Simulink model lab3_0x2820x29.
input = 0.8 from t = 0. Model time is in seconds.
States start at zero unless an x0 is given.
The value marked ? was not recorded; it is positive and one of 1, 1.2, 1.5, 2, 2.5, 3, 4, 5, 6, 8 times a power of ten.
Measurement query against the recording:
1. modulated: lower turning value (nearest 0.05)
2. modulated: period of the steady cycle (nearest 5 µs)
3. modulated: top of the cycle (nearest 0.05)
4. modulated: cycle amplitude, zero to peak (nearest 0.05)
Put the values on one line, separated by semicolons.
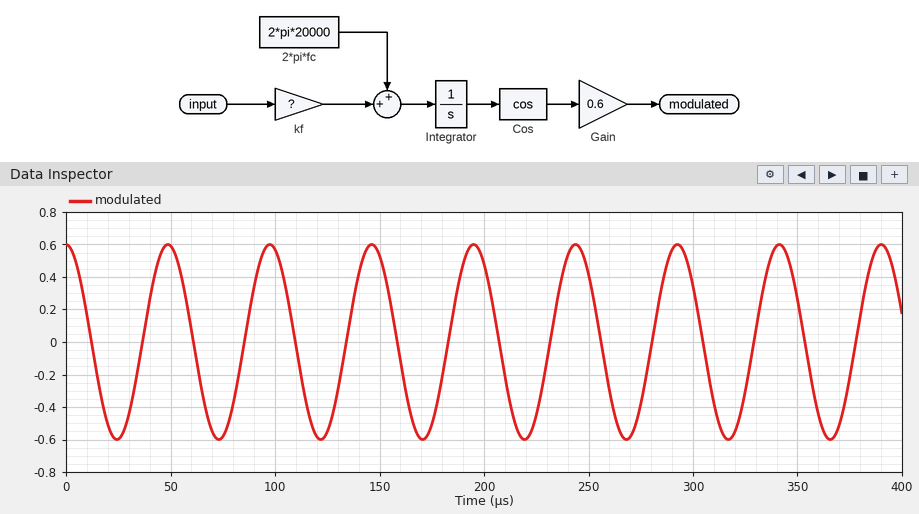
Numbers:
-0.60; 50 µs; 0.60; 0.60
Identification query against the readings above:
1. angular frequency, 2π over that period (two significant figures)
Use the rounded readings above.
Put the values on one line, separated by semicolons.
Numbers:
0.13 rad/µs
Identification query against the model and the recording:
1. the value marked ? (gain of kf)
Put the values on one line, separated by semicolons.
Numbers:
4000
